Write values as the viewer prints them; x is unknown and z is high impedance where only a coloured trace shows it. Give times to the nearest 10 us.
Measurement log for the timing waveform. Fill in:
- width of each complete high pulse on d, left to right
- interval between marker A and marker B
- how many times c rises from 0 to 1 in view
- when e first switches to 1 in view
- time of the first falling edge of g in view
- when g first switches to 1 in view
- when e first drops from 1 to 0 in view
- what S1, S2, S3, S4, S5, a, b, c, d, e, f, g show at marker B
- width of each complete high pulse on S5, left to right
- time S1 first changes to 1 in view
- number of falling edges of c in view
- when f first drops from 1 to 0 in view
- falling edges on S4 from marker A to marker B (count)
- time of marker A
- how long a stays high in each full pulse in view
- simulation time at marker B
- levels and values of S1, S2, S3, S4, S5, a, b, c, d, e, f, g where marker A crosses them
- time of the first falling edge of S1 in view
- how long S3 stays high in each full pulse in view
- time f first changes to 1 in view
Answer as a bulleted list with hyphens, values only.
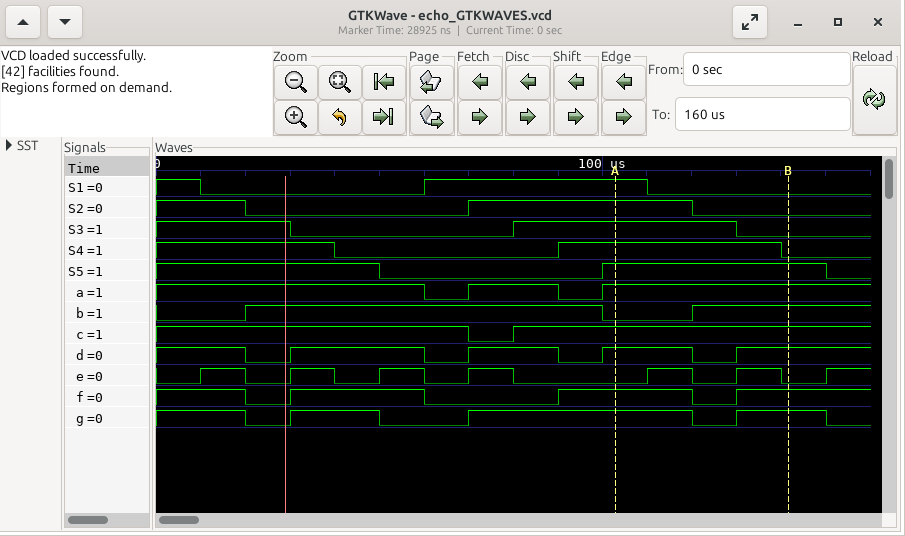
- 30 us, 20 us, 20 us
- 40 us
- 1
- 10 us
- 20 us
- 30 us
- 20 us
- S1=0, S2=0, S3=0, S4=0, S5=1, a=1, b=1, c=1, d=1, e=0, f=1, g=1
- 50 us
- 60 us
- 1
- 20 us
- 1
- 100 us
- 20 us
- 140 us
- S1=1, S2=1, S3=1, S4=1, S5=1, a=1, b=0, c=1, d=1, e=0, f=1, g=1
- 10 us
- 50 us
- 30 us
